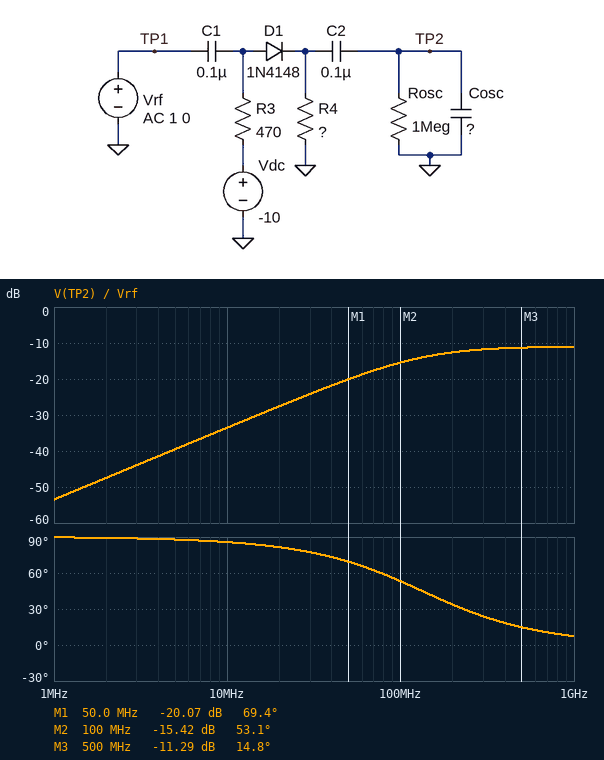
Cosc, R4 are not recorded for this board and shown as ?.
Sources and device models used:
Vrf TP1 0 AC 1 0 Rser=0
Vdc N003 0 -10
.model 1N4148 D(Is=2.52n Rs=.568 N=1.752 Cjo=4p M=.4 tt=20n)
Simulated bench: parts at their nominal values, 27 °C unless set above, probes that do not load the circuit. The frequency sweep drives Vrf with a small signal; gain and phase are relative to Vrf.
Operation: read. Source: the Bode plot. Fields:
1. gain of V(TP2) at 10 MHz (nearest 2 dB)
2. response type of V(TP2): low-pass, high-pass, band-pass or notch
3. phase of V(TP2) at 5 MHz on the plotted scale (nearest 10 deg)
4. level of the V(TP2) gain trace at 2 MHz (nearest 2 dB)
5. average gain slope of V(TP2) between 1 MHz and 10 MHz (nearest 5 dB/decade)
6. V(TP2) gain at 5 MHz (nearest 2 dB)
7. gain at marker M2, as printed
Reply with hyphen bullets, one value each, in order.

- -34 dB
- high-pass
- 90 deg
- -48 dB
- 20 dB/decade
- -40 dB
- -15.42 dB
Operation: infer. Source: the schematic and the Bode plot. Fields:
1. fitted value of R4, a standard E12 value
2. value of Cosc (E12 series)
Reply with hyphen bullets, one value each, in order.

- 220 Ω
- 3.9 pF
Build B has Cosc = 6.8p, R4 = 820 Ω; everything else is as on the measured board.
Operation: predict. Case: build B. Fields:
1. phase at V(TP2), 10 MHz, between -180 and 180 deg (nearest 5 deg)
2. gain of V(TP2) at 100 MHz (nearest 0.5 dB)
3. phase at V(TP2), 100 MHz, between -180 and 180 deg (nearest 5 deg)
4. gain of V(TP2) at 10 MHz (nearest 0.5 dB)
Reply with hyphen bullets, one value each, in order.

- 65 deg
- -15.0 dB
- 15 deg
- -23.0 dB
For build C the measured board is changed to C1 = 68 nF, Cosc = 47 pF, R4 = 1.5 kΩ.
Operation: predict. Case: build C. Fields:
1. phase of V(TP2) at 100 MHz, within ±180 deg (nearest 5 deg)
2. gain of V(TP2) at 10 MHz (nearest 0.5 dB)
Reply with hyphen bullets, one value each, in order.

- 0 deg
- -30.0 dB
